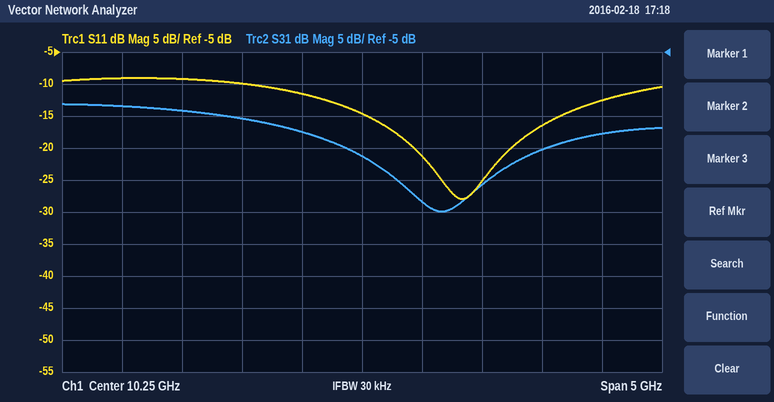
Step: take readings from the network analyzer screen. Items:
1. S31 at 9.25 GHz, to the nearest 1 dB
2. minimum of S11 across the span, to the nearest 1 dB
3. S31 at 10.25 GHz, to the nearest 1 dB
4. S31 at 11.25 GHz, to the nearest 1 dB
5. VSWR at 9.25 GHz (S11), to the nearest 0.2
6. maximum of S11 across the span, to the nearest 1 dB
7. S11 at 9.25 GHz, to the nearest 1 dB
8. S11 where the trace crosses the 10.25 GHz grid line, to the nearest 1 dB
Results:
-15 dB
-28 dB
-21 dB
-26 dB
2.0
-9 dB
-10 dB
-15 dB
